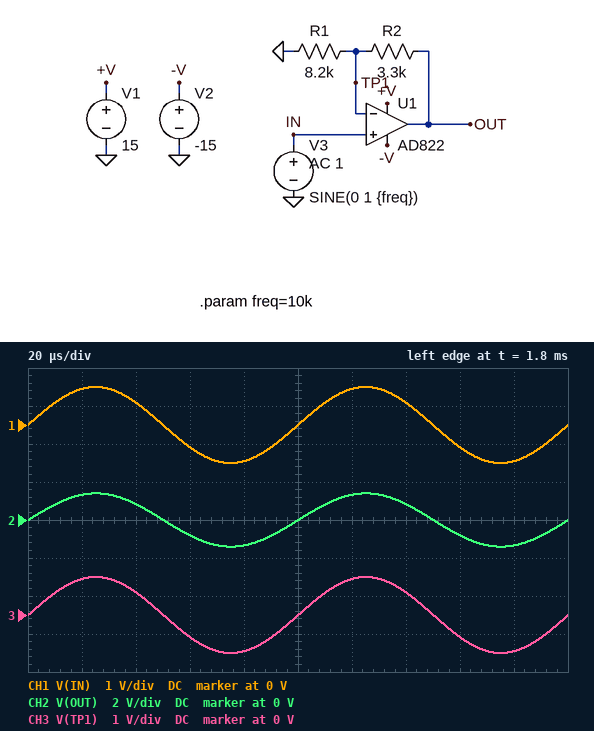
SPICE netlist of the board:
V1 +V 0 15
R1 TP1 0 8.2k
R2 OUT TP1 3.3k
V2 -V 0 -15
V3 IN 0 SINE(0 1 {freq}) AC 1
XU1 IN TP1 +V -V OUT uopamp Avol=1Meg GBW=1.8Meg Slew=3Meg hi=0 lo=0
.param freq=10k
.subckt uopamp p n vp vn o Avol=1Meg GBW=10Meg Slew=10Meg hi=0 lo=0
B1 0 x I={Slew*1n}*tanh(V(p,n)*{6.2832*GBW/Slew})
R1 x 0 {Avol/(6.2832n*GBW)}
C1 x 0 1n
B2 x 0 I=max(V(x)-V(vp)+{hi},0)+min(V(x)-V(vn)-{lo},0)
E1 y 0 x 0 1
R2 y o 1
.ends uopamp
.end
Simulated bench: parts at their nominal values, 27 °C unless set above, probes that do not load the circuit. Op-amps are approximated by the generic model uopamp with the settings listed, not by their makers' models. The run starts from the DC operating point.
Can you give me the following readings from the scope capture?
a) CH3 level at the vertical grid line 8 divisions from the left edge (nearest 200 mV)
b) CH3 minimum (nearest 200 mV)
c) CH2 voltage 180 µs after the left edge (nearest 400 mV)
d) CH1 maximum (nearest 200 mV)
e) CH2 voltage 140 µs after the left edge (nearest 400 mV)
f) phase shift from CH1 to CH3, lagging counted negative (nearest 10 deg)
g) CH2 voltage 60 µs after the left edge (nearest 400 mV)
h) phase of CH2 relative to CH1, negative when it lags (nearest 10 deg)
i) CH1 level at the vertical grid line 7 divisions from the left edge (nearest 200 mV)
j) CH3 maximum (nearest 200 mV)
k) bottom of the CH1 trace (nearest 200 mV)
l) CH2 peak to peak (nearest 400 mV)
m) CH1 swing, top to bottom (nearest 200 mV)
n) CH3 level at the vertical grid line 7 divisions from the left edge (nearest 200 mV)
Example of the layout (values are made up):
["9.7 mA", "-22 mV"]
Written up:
["-600 mV", "-1.0 V", "-1.2 V", "1.0 V", "800 mV", "0 deg", "-800 mV", "0 deg", "600 mV", "1.0 V", "-1.0 V", "2.8 V", "2.0 V", "600 mV"]
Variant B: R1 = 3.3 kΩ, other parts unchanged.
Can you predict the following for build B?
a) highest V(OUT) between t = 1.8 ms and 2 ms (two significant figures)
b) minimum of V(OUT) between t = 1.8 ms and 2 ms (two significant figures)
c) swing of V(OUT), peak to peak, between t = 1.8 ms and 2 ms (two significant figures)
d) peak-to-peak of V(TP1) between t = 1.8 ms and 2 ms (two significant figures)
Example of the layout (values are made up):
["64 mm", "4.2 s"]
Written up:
["2.0 V", "-2.0 V", "4.0 V", "2.0 V"]
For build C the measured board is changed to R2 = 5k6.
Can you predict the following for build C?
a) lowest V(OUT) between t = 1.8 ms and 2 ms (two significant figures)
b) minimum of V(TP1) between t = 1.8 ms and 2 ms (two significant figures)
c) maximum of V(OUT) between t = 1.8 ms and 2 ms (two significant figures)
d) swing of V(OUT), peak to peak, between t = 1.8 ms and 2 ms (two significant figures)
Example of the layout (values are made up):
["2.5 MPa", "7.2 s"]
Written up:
["-1.7 V", "-1.0 V", "1.7 V", "3.4 V"]
